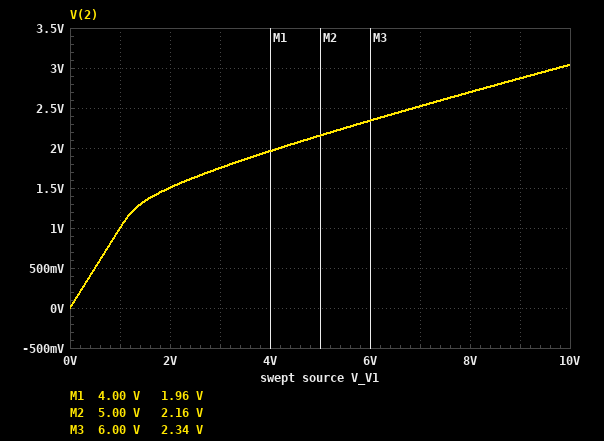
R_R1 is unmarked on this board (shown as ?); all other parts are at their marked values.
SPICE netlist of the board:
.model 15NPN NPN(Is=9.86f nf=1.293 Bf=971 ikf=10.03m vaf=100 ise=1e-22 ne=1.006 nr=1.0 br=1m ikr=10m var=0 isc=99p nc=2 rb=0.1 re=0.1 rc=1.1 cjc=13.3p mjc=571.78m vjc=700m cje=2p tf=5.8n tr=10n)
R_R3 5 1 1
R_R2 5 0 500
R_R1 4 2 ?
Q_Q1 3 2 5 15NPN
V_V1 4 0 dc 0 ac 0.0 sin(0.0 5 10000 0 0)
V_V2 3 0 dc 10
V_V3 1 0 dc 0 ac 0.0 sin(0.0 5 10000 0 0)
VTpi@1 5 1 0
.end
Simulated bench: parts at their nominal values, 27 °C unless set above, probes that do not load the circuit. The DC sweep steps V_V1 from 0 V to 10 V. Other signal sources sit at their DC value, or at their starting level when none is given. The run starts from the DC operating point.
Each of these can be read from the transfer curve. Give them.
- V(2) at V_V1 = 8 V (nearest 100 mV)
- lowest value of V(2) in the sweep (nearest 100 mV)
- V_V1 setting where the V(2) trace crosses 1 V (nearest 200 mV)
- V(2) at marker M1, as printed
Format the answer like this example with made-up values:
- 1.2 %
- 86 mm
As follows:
- 2.7 V
- 0 V
- 1.0 V
- 1.96 V
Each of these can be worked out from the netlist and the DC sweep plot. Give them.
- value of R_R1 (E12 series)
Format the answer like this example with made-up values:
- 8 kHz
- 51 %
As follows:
- 1.2 Ω
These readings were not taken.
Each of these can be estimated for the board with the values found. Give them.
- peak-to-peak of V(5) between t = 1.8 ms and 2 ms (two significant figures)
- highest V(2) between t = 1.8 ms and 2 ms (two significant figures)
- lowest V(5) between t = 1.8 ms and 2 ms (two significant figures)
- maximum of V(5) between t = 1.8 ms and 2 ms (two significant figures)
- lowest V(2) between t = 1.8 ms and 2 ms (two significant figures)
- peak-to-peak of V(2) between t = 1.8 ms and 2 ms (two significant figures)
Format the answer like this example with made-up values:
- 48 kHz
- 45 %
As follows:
- 10 V
- 5.0 V
- -5.0 V
- 5.0 V
- -5.0 V
- 10 V
